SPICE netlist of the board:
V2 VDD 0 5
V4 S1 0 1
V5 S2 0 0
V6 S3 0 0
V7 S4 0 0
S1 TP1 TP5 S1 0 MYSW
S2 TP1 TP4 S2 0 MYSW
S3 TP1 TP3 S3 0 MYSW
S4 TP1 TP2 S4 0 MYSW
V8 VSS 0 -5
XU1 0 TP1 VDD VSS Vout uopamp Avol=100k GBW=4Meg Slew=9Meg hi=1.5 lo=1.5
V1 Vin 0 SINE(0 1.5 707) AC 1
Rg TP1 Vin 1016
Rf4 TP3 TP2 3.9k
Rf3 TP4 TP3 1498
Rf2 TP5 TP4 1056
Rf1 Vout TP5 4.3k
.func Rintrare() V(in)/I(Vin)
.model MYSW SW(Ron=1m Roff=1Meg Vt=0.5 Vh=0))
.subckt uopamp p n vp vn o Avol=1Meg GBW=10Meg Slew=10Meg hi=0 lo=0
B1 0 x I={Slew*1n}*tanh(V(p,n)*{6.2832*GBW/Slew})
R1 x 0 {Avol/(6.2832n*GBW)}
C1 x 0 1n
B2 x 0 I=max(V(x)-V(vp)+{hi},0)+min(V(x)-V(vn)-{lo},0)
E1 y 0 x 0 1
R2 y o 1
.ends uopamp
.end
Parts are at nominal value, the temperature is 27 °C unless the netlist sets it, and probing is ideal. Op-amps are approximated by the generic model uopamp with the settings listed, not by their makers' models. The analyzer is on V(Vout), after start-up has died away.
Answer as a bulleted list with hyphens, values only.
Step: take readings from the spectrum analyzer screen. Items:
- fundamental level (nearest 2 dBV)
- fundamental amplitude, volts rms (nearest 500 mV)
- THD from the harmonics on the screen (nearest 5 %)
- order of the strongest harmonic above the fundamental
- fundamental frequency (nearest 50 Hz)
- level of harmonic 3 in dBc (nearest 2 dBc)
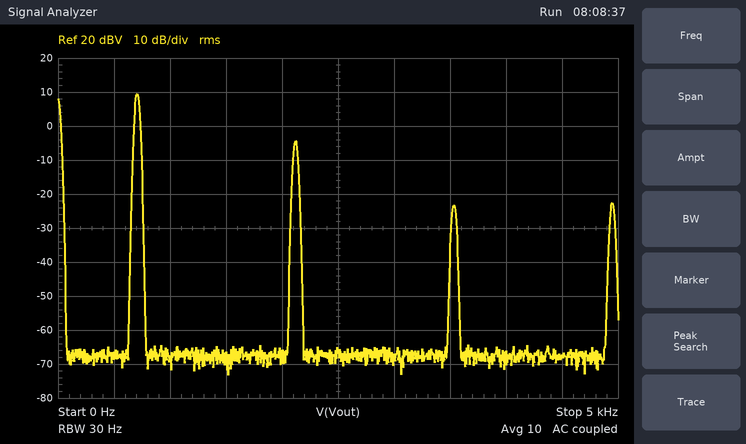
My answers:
- 10 dBV
- 3.0 V
- 20 %
- 3
- 700 Hz
- -14 dBc
